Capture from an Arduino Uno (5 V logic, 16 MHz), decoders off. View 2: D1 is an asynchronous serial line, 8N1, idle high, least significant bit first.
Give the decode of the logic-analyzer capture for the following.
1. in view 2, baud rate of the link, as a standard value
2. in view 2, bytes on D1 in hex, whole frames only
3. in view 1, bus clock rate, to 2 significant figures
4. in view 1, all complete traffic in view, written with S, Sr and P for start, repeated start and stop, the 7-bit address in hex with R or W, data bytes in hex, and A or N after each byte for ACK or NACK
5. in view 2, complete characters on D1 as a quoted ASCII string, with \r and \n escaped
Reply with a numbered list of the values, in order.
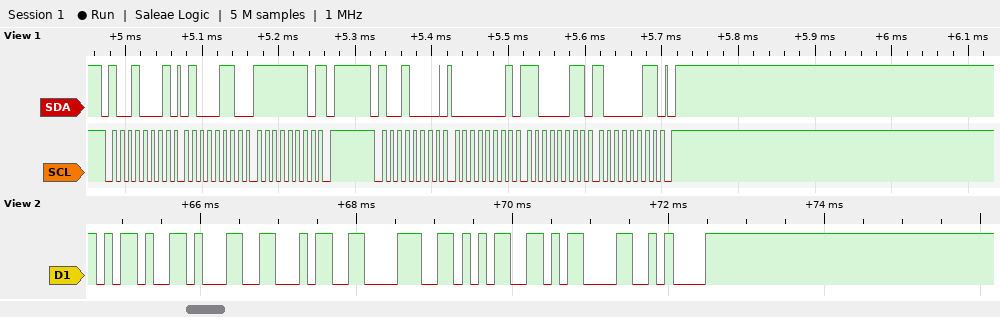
1. 9600 baud
2. 2D 31 34 38 35 0D 0A
3. 100 kHz
4. S 48R A 46 A FE N P S 48W A 01 A C3 A 83 A P
5. "-1485\r\n"
